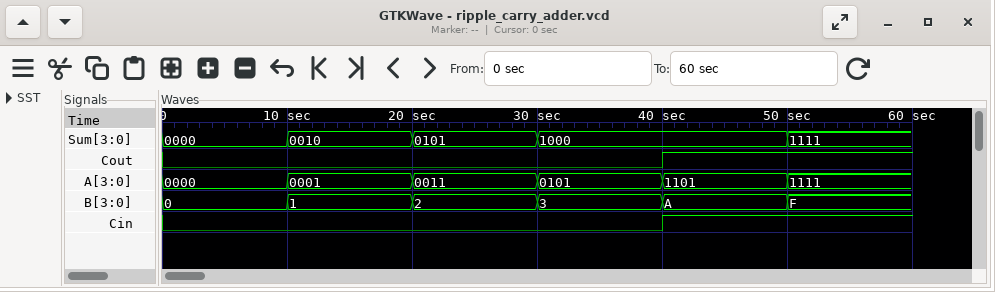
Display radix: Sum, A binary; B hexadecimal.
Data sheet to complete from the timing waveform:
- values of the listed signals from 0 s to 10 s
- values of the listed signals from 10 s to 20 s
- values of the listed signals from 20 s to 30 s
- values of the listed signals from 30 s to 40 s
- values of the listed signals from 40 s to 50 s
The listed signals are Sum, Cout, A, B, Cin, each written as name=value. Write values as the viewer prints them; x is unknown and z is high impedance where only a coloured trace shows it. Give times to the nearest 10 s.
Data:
Sum=0000, Cout=0, A=0000, B=0, Cin=0
Sum=0010, Cout=0, A=0001, B=1, Cin=0
Sum=0101, Cout=0, A=0011, B=2, Cin=0
Sum=1000, Cout=0, A=0101, B=3, Cin=0
Sum=1000, Cout=1, A=1101, B=A, Cin=1
